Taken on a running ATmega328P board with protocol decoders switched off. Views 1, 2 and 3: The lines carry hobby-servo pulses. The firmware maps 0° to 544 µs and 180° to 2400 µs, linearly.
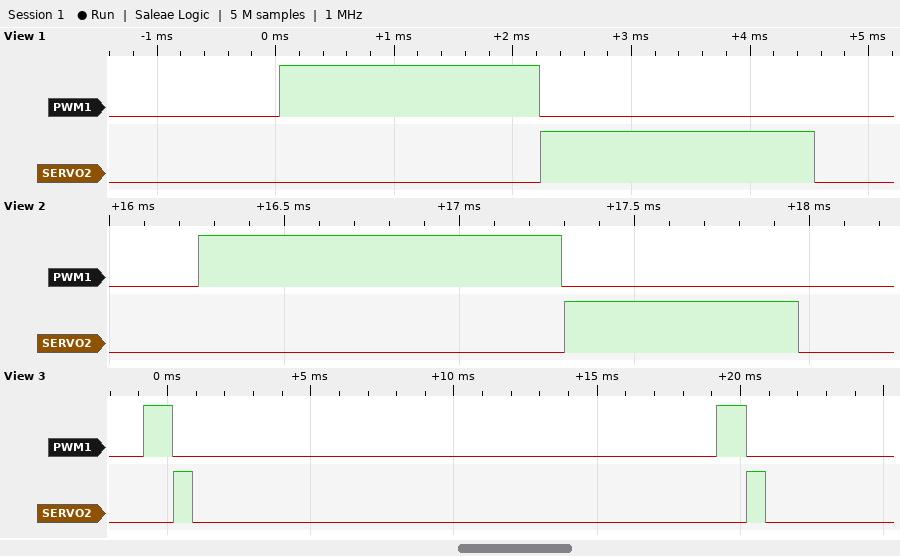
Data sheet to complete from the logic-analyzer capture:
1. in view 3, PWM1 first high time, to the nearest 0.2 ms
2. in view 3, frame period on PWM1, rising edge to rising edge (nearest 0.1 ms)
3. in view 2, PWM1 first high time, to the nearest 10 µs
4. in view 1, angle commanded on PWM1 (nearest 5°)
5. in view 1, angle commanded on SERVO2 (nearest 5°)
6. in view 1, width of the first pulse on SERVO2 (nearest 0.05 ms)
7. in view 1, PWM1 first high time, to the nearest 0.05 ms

1.0 ms
20.0 ms
1040 µs
160°
170°
2.30 ms
2.20 ms
